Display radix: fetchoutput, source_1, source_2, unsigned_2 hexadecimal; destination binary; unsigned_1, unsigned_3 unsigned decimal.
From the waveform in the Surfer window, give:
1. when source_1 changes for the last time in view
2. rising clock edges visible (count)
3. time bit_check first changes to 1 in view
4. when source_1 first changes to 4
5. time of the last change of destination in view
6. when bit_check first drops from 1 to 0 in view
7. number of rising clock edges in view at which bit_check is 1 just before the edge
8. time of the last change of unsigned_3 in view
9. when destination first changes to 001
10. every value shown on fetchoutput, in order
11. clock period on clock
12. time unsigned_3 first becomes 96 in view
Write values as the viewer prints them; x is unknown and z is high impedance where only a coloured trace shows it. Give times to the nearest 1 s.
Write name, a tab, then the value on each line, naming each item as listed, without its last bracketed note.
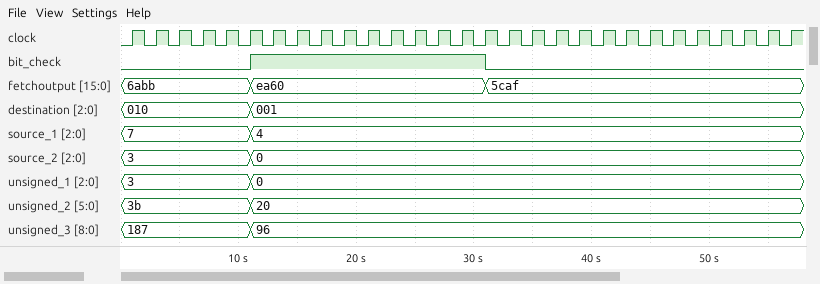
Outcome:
when source_1 changes for the last time in view	11 s
rising clock edges visible	29
time bit_check first changes to 1 in view	11 s
when source_1 first changes to 4	11 s
time of the last change of destination in view	11 s
when bit_check first drops from 1 to 0 in view	31 s
number of rising clock edges in view at which bit_check is 1 just before the edge	10
time of the last change of unsigned_3 in view	11 s
when destination first changes to 001	11 s
every value shown on fetchoutput, in order	6abb, ea60, 5caf
clock period on clock	2 s
time unsigned_3 first becomes 96 in view	11 s
